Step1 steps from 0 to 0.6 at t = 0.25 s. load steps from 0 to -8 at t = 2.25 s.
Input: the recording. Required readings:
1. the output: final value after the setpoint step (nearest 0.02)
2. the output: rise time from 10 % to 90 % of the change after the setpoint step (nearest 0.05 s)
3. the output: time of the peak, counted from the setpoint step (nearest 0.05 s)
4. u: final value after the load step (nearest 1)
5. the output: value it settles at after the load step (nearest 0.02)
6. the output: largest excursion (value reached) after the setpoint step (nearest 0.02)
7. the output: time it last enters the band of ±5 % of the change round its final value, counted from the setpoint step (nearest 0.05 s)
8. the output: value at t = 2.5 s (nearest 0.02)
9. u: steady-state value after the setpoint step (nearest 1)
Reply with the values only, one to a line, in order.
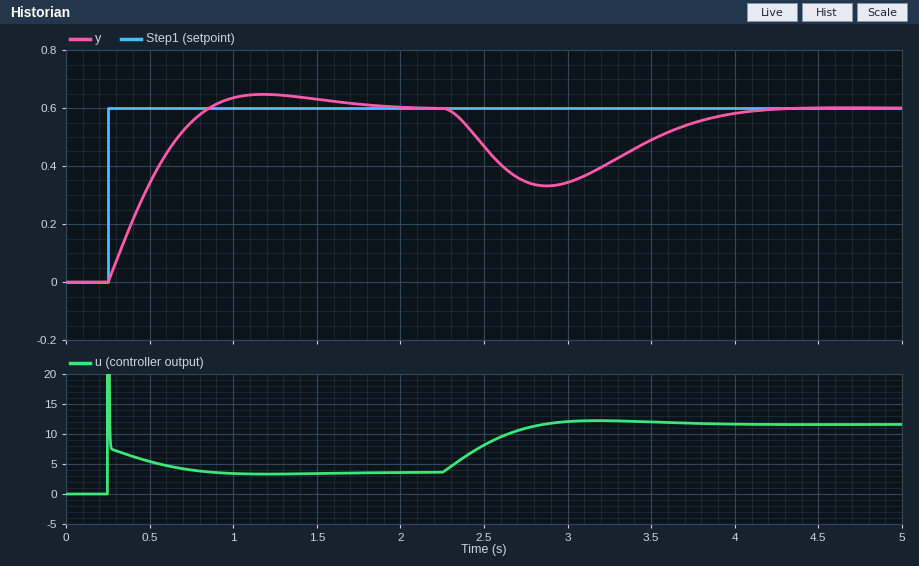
0.60
0.45 s
0.95 s
12
0.60
0.64
1.25 s
0.46
4
